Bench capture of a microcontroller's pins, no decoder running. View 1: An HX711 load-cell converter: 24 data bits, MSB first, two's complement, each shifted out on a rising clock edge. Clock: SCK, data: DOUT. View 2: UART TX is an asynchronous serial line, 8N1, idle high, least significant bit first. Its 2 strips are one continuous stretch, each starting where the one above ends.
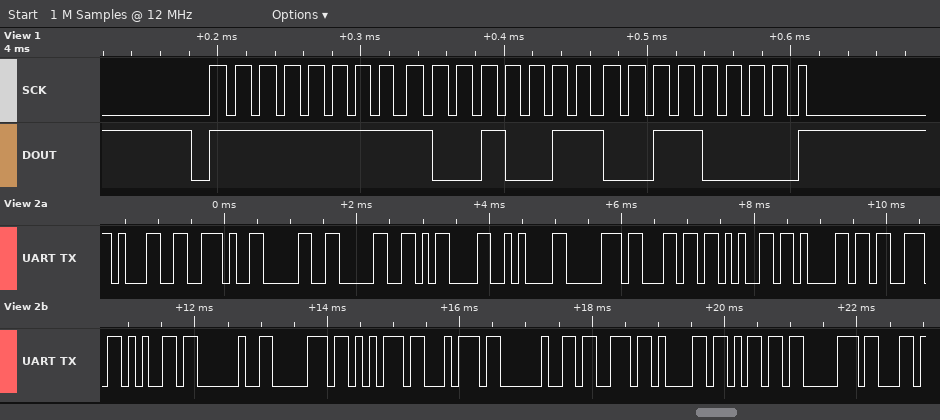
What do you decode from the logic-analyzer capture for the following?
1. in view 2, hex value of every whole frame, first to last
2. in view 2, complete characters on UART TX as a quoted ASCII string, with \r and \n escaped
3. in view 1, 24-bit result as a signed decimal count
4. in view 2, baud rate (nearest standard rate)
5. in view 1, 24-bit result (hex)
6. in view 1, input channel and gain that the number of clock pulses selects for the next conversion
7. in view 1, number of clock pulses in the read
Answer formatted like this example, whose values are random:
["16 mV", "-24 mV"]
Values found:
["31 2E 30 30 0D 0A 70 6C 65 61 73 65 20 70 75 74 20 73 61 6D 70", "\"1.00\\r\\nplease put samp\"", "-27856", "9600 baud", "0xFF9330", "channel A, gain 128", "25"]
